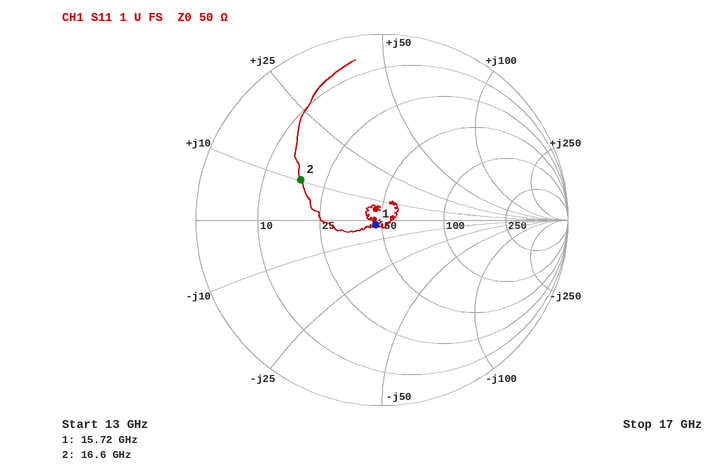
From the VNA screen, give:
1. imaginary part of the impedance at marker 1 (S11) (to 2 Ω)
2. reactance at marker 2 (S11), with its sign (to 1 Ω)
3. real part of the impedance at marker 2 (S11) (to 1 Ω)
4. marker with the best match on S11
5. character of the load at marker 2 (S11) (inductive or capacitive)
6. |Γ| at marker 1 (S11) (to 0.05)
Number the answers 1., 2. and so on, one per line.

1. -2 Ω
2. +10 Ω
3. 18 Ω
4. marker 1
5. inductive
6. 0.05
